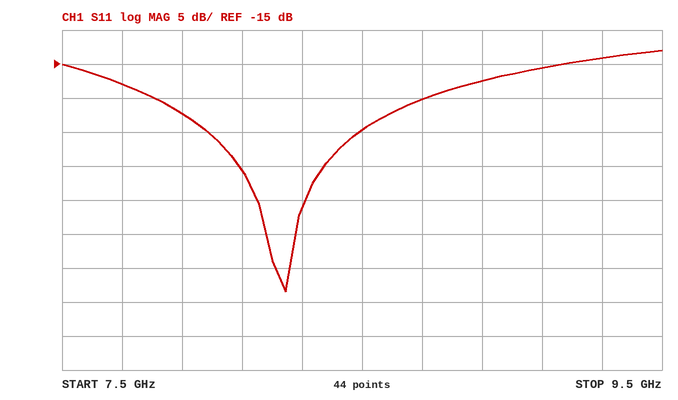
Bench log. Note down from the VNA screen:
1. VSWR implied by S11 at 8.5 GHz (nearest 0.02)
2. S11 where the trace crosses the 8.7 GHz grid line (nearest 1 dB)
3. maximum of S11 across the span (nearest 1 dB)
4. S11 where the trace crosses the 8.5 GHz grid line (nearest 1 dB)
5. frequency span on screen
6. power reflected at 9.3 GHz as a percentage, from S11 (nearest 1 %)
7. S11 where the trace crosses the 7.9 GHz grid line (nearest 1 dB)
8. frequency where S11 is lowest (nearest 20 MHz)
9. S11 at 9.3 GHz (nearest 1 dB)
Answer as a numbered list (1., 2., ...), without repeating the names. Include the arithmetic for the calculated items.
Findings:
1. |Γ| = 10^(-25/20) = 0.0562; VSWR = (1 + 0.0562)/(1 − 0.0562) ≈ 1.12
2. -20 dB
3. -13 dB
4. -25 dB
5. 2 GHz
6. 10^(-14/10) ≈ 4 %
7. -22 dB
8. 8.24 GHz
9. -14 dB
